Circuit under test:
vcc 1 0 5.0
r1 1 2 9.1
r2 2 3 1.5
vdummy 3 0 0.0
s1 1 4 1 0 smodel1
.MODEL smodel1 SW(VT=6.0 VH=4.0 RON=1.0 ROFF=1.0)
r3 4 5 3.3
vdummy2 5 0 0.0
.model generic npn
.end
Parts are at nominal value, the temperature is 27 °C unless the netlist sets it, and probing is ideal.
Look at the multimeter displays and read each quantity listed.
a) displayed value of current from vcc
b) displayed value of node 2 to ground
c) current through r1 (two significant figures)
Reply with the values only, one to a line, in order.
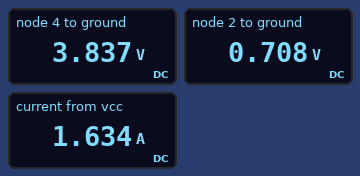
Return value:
1.634 A
0.708 V
470 mA
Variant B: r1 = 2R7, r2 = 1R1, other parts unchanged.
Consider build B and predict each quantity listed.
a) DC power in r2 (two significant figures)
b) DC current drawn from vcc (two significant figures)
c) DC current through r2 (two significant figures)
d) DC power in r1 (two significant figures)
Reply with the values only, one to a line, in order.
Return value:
1.9 W
2.5 A
1.3 A
4.7 W
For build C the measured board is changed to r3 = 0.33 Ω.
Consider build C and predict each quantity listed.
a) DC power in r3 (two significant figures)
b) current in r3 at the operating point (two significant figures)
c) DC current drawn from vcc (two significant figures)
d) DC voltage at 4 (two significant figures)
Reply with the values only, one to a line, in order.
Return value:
4.7 W
3.8 A
4.2 A
1.2 V
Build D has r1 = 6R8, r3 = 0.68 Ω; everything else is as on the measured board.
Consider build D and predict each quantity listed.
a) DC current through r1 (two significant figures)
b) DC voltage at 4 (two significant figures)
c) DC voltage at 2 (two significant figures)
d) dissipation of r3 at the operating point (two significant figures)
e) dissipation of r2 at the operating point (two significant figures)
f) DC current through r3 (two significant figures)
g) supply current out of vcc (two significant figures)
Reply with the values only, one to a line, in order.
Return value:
600 mA
2.0 V
900 mV
6.0 W
540 mW
3.0 A
3.6 A
